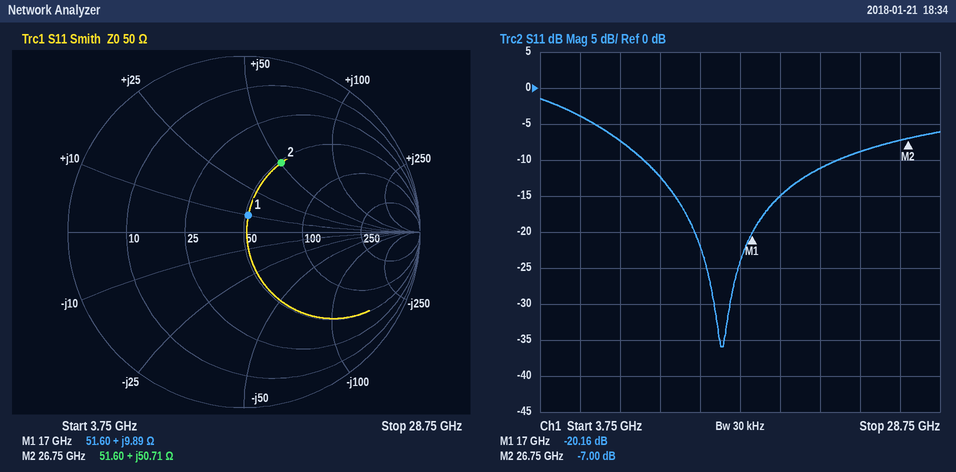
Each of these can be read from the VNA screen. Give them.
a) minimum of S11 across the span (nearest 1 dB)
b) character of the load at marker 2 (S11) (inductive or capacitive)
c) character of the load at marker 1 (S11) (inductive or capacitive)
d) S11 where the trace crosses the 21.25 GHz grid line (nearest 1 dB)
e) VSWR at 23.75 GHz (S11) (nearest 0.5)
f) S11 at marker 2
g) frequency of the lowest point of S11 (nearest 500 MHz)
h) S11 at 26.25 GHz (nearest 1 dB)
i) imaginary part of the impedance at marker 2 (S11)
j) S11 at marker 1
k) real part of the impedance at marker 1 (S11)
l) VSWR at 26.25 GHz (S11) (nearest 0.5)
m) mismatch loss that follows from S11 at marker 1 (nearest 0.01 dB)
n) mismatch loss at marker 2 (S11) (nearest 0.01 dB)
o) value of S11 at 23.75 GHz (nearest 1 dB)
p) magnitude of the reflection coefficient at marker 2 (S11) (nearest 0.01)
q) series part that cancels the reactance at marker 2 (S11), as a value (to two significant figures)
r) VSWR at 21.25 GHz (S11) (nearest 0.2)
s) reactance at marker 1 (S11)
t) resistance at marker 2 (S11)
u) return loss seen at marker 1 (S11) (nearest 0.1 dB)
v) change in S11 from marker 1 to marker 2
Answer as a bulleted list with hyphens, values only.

- -36 dB
- inductive
- inductive
- -11 dB
- 2.0
- -7.00 dB
- 15.0 GHz
- -7 dB
- +50.71 Ω
- -20.16 dB
- 51.60 Ω
- 2.5
- 0.04 dB
- 0.97 dB
- -9 dB
- 0.45
- 120 fF
- 1.8
- +9.89 Ω
- 51.60 Ω
- 20.2 dB
- 13.16 dB
